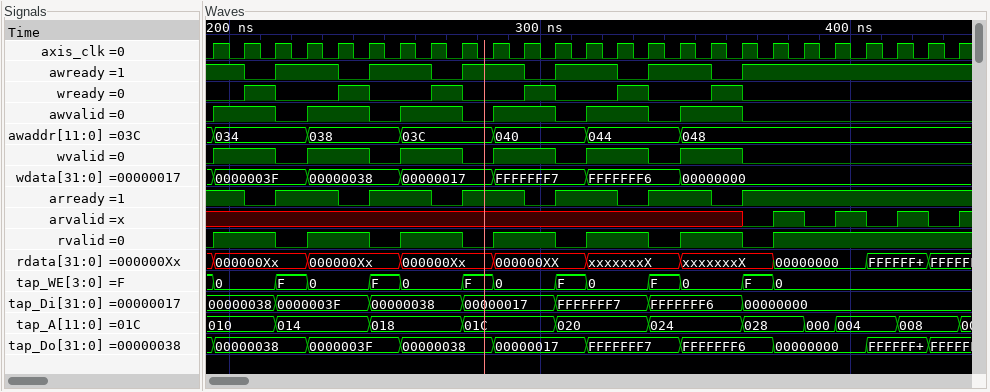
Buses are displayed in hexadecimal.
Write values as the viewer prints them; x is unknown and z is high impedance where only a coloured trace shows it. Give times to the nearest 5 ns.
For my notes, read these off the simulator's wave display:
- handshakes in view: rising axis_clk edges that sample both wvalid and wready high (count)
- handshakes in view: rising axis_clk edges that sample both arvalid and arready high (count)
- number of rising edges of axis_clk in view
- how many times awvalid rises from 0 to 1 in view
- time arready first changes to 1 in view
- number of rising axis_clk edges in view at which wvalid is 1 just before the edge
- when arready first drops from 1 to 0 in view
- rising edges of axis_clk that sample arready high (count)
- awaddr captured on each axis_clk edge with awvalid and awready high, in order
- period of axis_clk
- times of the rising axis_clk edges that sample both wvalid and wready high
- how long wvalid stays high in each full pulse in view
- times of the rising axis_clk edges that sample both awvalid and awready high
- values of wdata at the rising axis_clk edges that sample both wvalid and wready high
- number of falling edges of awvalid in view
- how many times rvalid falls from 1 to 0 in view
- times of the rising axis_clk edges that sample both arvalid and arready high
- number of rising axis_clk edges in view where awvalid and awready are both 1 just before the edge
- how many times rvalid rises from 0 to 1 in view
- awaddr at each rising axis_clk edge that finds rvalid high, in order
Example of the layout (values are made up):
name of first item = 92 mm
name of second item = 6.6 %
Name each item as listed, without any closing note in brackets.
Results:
handshakes in view: rising axis_clk edges that sample both wvalid and wready high = 6
handshakes in view: rising axis_clk edges that sample both arvalid and arready high = 3
number of rising edges of axis_clk in view = 25
how many times awvalid rises from 0 to 1 in view = 6
time arready first changes to 1 in view = 215 ns
number of rising axis_clk edges in view at which wvalid is 1 just before the edge = 12
when arready first drops from 1 to 0 in view = 205 ns
rising edges of axis_clk that sample arready high = 19
awaddr captured on each axis_clk edge with awvalid and awready high, in order = 034, 038, 03C, 040, 044, 048
period of axis_clk = 10 ns
times of the rising axis_clk edges that sample both wvalid and wready high = 215 ns, 245 ns, 275 ns, 305 ns, 335 ns, 365 ns
how long wvalid stays high in each full pulse in view = 20 ns, 20 ns, 20 ns, 20 ns, 20 ns, 20 ns
times of the rising axis_clk edges that sample both awvalid and awready high = 205 ns, 235 ns, 265 ns, 295 ns, 325 ns, 355 ns
values of wdata at the rising axis_clk edges that sample both wvalid and wready high = 0000003F, 00000038, 00000017, FFFFFFF7, FFFFFFF6, 00000000
number of falling edges of awvalid in view = 6
how many times rvalid falls from 1 to 0 in view = 6
times of the rising axis_clk edges that sample both arvalid and arready high = 385 ns, 405 ns, 425 ns
number of rising axis_clk edges in view where awvalid and awready are both 1 just before the edge = 6
how many times rvalid rises from 0 to 1 in view = 7
awaddr at each rising axis_clk edge that finds rvalid high, in order = 034, 034, 038, 038, 03C, 03C, 040, 040, 044, 044, 048, 048, 048, 048, 048, 048, 048, 048
